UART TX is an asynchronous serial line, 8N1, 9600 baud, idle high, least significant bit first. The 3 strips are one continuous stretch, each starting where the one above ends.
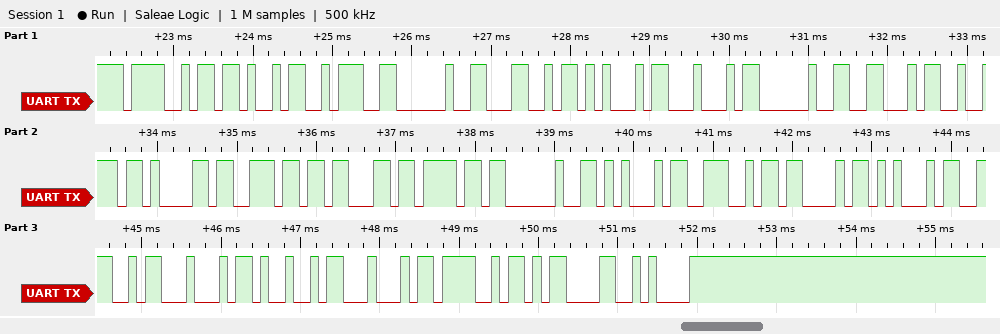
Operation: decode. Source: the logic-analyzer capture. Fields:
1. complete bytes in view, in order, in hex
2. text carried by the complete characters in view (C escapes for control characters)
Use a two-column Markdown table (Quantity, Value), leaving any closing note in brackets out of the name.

| Quantity | Value |
|---|---|
| complete bytes in view, in order, in hex | 4F 4B 3A 20 4C 45 44 20 46 72 61 6E 63 6F 20 45 4E 43 45 4E 44 49 44 4F 0D 0A |
| text carried by the complete characters in view | "OK: LED Franco ENCENDIDO\r\n" |
